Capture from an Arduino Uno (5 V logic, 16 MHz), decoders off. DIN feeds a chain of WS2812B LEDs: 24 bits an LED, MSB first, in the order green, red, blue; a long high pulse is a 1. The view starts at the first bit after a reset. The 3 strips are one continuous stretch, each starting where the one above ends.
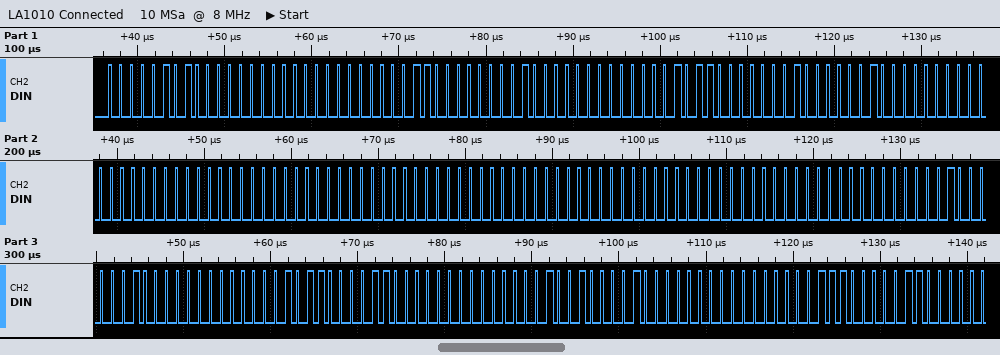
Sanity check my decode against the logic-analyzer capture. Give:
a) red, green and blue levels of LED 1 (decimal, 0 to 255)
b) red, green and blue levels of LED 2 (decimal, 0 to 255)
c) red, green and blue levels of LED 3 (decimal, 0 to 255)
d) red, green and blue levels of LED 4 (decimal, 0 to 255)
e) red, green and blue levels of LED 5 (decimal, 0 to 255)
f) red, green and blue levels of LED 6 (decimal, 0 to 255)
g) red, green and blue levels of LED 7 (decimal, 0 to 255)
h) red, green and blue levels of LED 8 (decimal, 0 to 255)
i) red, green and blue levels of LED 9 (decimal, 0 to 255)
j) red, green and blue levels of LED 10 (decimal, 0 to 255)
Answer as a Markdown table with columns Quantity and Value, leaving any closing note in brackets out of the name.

| Quantity | Value |
|---|---|
| red, green and blue levels of LED 1 | 0, 5, 0 |
| red, green and blue levels of LED 2 | 2, 12, 0 |
| red, green and blue levels of LED 3 | 1, 11, 2 |
| red, green and blue levels of LED 4 | 0, 0, 0 |
| red, green and blue levels of LED 5 | 0, 0, 0 |
| red, green and blue levels of LED 6 | 0, 0, 0 |
| red, green and blue levels of LED 7 | 1, 0, 2 |
| red, green and blue levels of LED 8 | 11, 0, 12 |
| red, green and blue levels of LED 9 | 9, 0, 8 |
| red, green and blue levels of LED 10 | 7, 0, 6 |
